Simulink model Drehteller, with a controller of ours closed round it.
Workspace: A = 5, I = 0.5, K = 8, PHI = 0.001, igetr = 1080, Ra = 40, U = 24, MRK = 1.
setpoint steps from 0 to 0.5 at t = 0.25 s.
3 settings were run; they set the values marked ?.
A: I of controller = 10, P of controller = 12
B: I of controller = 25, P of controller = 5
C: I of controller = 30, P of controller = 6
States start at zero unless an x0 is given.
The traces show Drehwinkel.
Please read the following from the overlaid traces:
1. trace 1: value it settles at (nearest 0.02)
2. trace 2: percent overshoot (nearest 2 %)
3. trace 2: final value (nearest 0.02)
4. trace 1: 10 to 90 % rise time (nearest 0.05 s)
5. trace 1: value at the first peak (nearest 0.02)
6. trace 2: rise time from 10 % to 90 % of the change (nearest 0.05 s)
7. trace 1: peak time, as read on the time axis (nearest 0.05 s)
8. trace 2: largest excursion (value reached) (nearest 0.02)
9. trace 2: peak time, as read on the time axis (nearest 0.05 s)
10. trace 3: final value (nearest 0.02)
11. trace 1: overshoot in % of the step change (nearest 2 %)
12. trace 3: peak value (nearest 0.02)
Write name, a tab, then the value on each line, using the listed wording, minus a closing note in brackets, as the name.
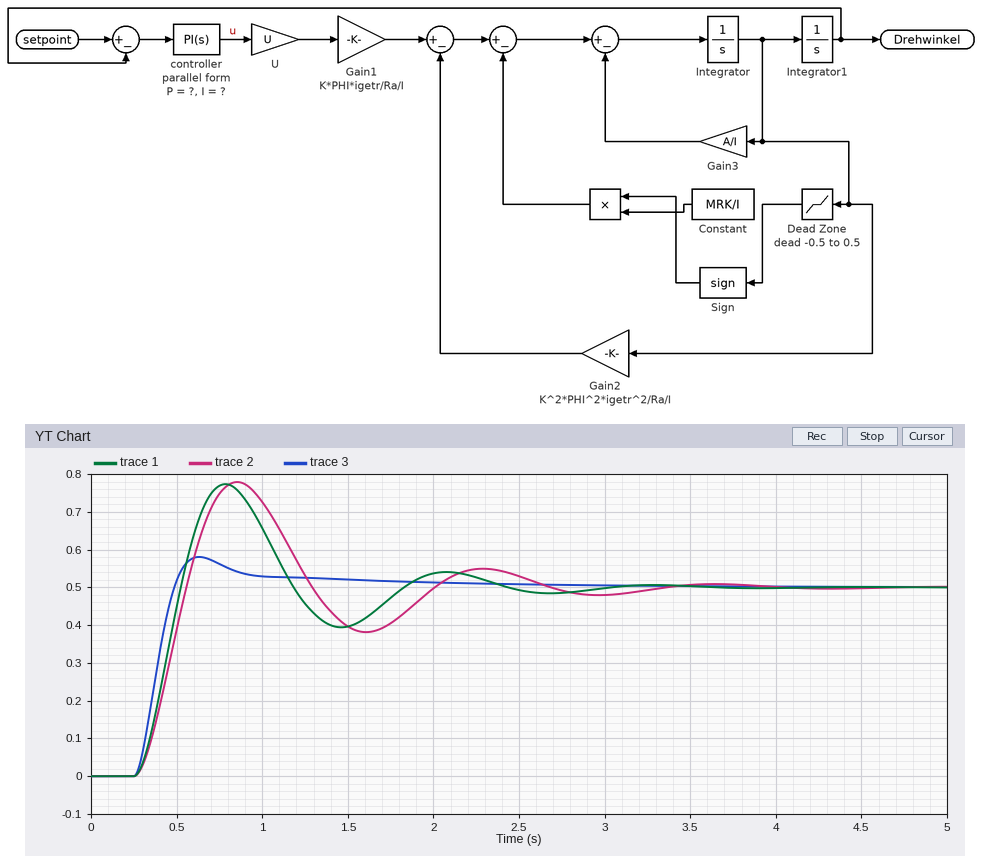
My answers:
trace 1: value it settles at	0.50
trace 2: percent overshoot	56 %
trace 2: final value	0.50
trace 1: 10 to 90 % rise time	0.20 s
trace 1: value at the first peak	0.78
trace 2: rise time from 10 % to 90 % of the change	0.20 s
trace 1: peak time, as read on the time axis	0.80 s
trace 2: largest excursion (value reached)	0.78
trace 2: peak time, as read on the time axis	0.85 s
trace 3: final value	0.50
trace 1: overshoot in % of the step change	54 %
trace 3: peak value	0.58
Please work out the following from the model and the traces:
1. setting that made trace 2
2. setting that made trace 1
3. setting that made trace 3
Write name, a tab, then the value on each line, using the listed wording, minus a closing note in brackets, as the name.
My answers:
setting that made trace 2	B
setting that made trace 1	C
setting that made trace 3	A
